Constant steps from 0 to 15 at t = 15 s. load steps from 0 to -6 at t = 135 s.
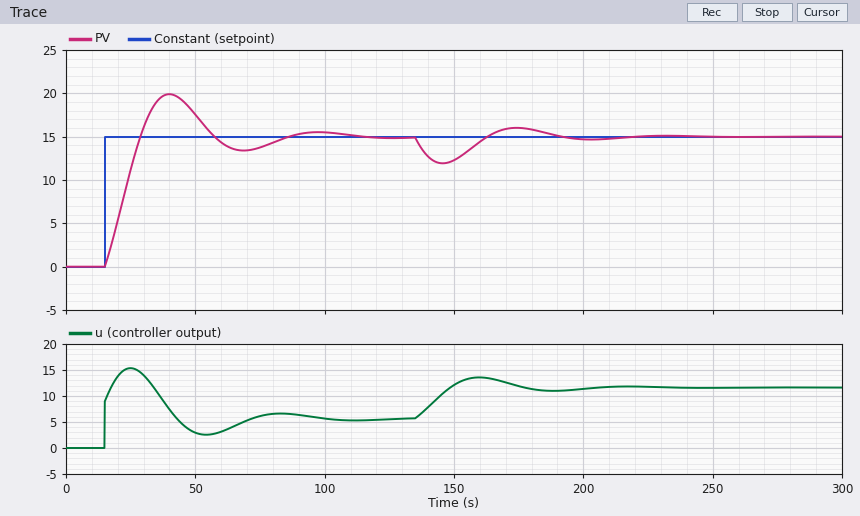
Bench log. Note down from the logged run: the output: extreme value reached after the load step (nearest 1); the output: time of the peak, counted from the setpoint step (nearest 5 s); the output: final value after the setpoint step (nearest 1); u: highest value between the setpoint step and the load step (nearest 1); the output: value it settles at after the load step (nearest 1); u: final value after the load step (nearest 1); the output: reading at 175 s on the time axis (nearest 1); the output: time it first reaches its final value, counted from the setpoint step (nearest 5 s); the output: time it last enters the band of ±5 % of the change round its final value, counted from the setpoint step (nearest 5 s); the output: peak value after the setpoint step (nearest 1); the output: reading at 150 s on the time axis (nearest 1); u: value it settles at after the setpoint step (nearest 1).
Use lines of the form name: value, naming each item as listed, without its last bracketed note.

the output: extreme value reached after the load step: 12
the output: time of the peak, counted from the setpoint step: 25 s
the output: final value after the setpoint step: 15
u: highest value between the setpoint step and the load step: 15
the output: value it settles at after the load step: 15
u: final value after the load step: 12
the output: reading at 175 s on the time axis: 16
the output: time it first reaches its final value, counted from the setpoint step: 15 s
the output: time it last enters the band of ±5 % of the change round its final value, counted from the setpoint step: 65 s
the output: peak value after the setpoint step: 20
the output: reading at 150 s on the time axis: 12
u: value it settles at after the setpoint step: 6
